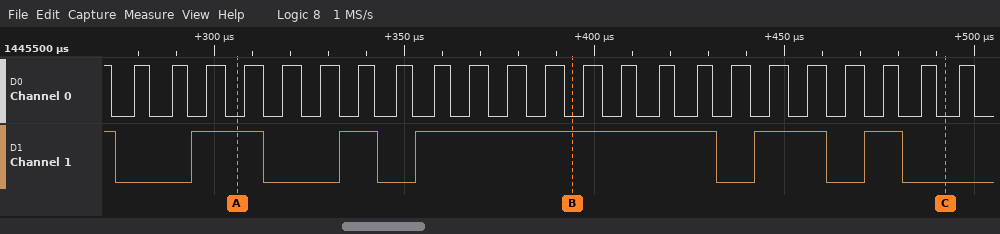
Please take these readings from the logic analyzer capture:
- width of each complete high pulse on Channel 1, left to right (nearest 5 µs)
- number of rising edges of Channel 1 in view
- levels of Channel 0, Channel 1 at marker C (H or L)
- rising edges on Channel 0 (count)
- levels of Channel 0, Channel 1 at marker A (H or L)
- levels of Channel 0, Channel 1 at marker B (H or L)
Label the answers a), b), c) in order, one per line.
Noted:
a) 20 µs, 10 µs, 80 µs, 20 µs, 10 µs
b) 5
c) Channel 0=L, Channel 1=L
d) 23
e) Channel 0=L, Channel 1=H
f) Channel 0=L, Channel 1=H
